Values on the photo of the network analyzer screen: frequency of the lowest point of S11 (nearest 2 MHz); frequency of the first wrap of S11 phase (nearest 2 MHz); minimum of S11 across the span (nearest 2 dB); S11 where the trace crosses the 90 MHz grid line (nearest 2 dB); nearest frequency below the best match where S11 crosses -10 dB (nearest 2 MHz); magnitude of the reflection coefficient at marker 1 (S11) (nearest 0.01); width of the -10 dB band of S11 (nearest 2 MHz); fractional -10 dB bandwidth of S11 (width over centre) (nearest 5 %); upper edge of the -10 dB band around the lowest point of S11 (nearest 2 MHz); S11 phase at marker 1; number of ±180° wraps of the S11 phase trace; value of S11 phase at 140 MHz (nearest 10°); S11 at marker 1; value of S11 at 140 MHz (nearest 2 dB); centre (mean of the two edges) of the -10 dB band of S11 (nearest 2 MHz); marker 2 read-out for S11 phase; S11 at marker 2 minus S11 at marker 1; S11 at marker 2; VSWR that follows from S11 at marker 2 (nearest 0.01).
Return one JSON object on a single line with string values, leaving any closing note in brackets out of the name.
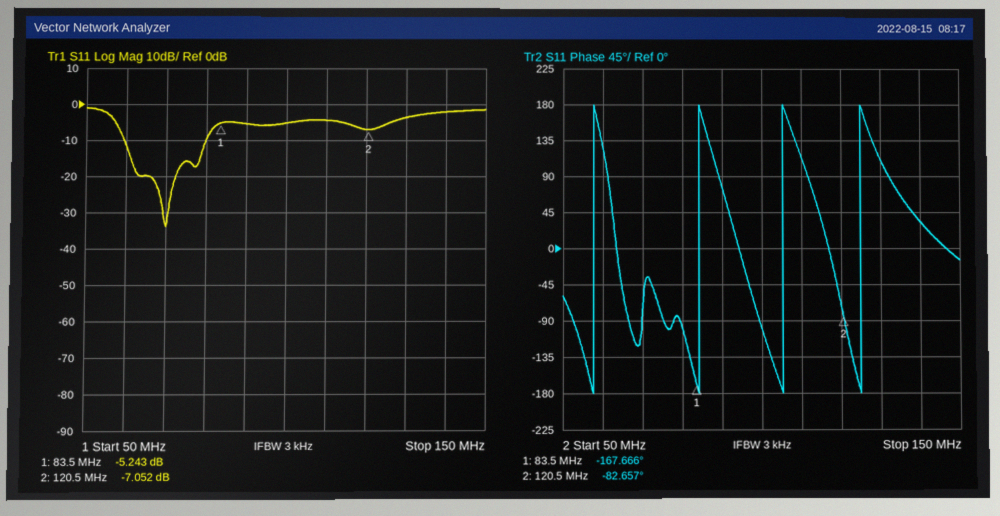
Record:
{"frequency of the lowest point of S11": "70 MHz", "frequency of the first wrap of S11 phase": "58 MHz", "minimum of S11 across the span": "-34 dB", "S11 where the trace crosses the 90 MHz grid line": "-6 dB", "nearest frequency below the best match where S11 crosses -10 dB": "60 MHz", "magnitude of the reflection coefficient at marker 1 (S11)": "0.55", "width of the -10 dB band of S11": "20 MHz", "fractional -10 dB bandwidth of S11 (width over centre)": "30 %", "upper edge of the -10 dB band around the lowest point of S11": "80 MHz", "S11 phase at marker 1": "-167.666°", "number of ±180° wraps of the S11 phase trace": "4", "value of S11 phase at 140 MHz": "30°", "S11 at marker 1": "-5.243 dB", "value of S11 at 140 MHz": "-2 dB", "centre (mean of the two edges) of the -10 dB band of S11": "70 MHz", "marker 2 read-out for S11 phase": "-82.657°", "S11 at marker 2 minus S11 at marker 1": "-1.809 dB", "S11 at marker 2": "-7.052 dB", "VSWR that follows from S11 at marker 2": "2.60"}
